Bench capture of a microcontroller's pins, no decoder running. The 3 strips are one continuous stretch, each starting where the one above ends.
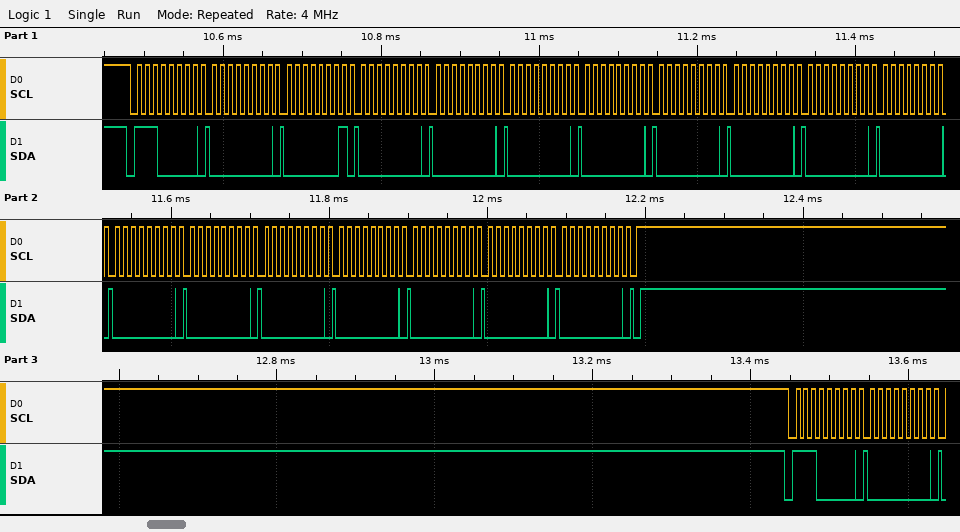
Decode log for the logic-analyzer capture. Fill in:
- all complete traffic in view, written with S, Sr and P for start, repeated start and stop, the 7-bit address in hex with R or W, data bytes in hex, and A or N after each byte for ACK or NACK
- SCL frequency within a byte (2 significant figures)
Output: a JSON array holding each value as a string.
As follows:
["S 70W A 00 A 01 A 00 A 00 A 00 A 00 A 00 A 00 A 00 A 00 A 00 A 00 A 00 A 00 A 00 A 00 A 00 A P S 70W A 00 A", "100 kHz"]
